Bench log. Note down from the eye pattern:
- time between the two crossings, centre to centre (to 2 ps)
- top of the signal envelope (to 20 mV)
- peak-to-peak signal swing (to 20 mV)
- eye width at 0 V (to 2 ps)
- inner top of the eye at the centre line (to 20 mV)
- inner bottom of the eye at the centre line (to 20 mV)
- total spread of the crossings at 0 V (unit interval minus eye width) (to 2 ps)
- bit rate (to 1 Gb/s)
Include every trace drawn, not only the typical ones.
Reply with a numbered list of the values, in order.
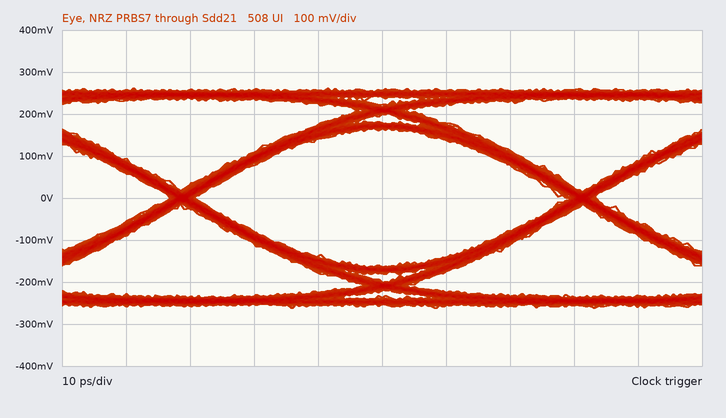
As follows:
1. 62 ps
2. 260 mV
3. 520 mV
4. 58 ps
5. 160 mV
6. -160 mV
7. 4 ps
8. 16 Gb/s
